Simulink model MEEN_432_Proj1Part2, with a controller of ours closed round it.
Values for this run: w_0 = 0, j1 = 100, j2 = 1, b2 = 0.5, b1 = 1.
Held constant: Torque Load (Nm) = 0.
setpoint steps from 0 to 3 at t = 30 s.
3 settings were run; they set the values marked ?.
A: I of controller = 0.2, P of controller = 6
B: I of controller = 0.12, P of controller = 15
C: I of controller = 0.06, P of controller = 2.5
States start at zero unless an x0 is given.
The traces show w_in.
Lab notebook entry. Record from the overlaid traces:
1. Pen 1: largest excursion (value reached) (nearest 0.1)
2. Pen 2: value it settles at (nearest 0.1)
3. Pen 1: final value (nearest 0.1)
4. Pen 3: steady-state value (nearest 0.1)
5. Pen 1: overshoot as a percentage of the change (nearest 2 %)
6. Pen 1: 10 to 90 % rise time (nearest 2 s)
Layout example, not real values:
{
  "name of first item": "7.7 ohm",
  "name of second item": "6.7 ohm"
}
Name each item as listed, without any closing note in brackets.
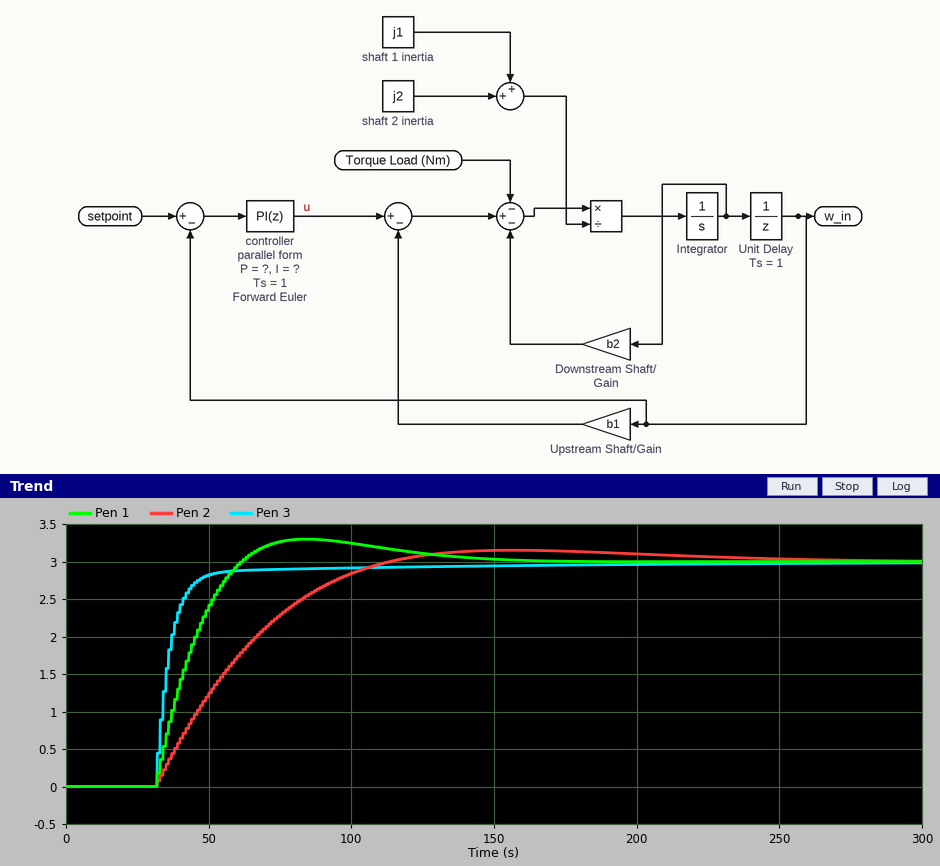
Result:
{
  "Pen 1: largest excursion (value reached)": "3.3",
  "Pen 2: value it settles at": "3.0",
  "Pen 1: final value": "3.0",
  "Pen 3: steady-state value": "3.0",
  "Pen 1: overshoot as a percentage of the change": "10 %",
  "Pen 1: 10 to 90 % rise time": "22 s"
}
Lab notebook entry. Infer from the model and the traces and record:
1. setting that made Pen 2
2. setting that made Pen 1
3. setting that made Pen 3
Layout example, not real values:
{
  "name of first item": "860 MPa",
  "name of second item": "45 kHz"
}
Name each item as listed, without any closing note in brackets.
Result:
{
  "setting that made Pen 2": "C",
  "setting that made Pen 1": "A",
  "setting that made Pen 3": "B"
}
